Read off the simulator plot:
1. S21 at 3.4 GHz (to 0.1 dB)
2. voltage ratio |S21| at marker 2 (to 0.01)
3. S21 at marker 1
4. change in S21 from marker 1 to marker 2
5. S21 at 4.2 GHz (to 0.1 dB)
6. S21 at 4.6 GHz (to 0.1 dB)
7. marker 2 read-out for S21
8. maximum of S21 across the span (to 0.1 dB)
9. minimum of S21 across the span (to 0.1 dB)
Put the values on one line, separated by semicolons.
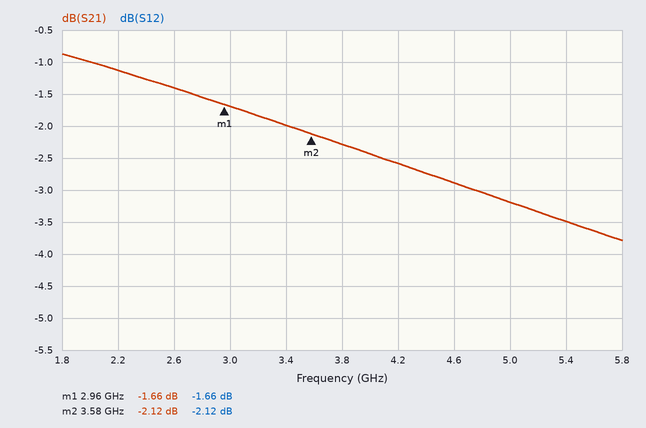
-2.0 dB; 0.78; -1.66 dB; -0.46 dB; -2.6 dB; -2.9 dB; -2.12 dB; -0.9 dB; -3.8 dB
